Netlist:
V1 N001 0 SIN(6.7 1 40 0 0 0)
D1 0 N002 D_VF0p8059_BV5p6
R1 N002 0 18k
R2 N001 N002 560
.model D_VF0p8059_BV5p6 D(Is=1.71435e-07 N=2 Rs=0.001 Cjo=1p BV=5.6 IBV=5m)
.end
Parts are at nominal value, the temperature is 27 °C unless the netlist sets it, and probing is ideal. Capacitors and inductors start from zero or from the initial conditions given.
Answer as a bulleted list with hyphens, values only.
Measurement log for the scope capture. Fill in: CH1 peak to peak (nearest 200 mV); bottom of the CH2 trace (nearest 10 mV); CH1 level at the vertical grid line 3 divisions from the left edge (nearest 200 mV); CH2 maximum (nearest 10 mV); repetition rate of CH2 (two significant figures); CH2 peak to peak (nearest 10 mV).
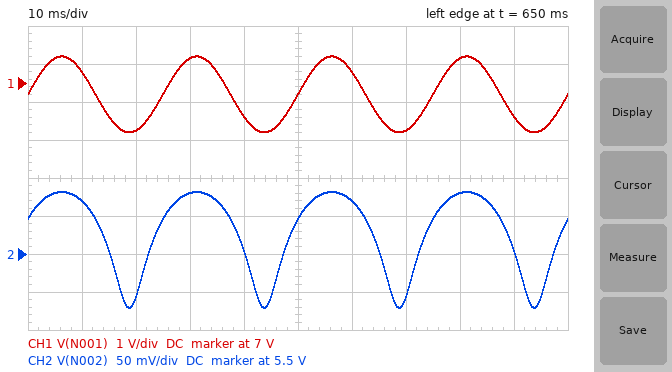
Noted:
- 2.0 V
- 5.43 V
- 7.6 V
- 5.58 V
- 40 Hz
- 150 mV
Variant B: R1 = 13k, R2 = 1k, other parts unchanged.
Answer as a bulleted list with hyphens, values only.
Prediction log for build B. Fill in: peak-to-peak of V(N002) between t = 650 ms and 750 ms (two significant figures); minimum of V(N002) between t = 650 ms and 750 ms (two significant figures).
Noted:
- 260 mV
- 5.3 V
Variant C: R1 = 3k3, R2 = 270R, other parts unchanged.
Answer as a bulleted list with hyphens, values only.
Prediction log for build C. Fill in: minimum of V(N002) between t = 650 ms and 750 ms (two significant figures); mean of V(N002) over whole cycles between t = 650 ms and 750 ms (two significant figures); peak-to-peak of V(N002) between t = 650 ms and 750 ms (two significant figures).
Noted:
- 5.3 V
- 5.5 V
- 340 mV
